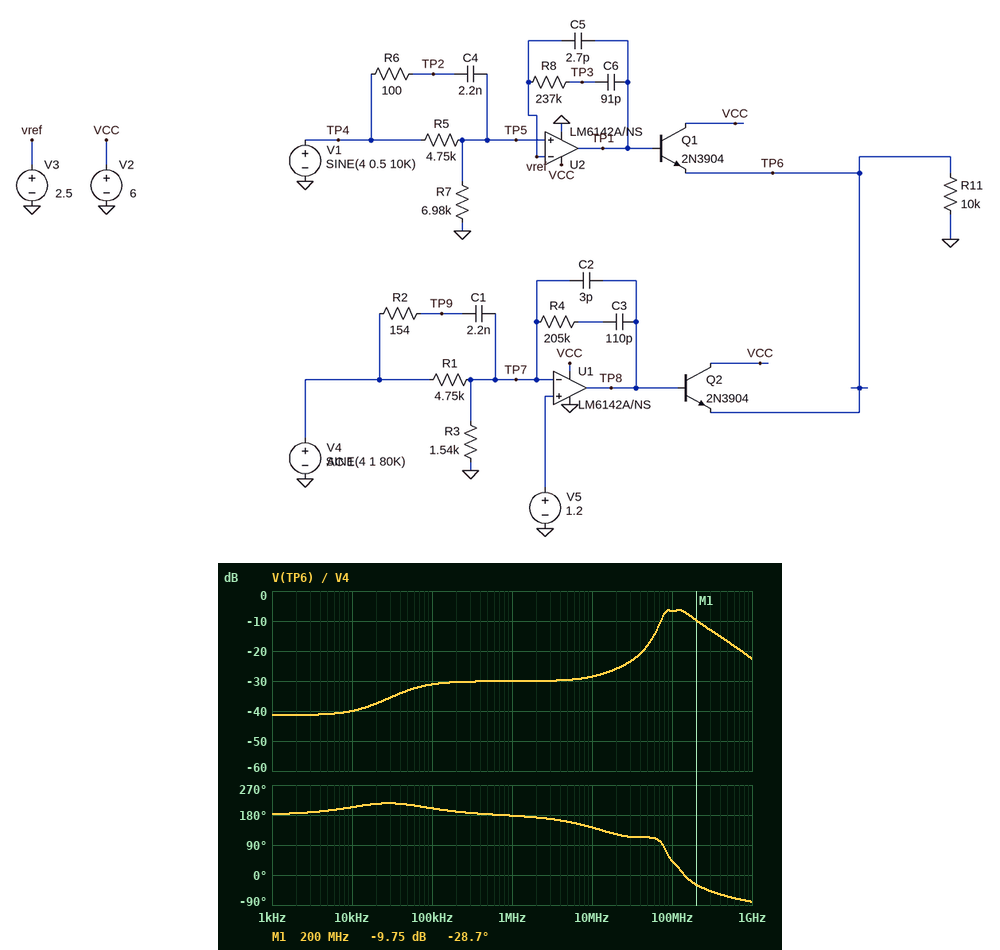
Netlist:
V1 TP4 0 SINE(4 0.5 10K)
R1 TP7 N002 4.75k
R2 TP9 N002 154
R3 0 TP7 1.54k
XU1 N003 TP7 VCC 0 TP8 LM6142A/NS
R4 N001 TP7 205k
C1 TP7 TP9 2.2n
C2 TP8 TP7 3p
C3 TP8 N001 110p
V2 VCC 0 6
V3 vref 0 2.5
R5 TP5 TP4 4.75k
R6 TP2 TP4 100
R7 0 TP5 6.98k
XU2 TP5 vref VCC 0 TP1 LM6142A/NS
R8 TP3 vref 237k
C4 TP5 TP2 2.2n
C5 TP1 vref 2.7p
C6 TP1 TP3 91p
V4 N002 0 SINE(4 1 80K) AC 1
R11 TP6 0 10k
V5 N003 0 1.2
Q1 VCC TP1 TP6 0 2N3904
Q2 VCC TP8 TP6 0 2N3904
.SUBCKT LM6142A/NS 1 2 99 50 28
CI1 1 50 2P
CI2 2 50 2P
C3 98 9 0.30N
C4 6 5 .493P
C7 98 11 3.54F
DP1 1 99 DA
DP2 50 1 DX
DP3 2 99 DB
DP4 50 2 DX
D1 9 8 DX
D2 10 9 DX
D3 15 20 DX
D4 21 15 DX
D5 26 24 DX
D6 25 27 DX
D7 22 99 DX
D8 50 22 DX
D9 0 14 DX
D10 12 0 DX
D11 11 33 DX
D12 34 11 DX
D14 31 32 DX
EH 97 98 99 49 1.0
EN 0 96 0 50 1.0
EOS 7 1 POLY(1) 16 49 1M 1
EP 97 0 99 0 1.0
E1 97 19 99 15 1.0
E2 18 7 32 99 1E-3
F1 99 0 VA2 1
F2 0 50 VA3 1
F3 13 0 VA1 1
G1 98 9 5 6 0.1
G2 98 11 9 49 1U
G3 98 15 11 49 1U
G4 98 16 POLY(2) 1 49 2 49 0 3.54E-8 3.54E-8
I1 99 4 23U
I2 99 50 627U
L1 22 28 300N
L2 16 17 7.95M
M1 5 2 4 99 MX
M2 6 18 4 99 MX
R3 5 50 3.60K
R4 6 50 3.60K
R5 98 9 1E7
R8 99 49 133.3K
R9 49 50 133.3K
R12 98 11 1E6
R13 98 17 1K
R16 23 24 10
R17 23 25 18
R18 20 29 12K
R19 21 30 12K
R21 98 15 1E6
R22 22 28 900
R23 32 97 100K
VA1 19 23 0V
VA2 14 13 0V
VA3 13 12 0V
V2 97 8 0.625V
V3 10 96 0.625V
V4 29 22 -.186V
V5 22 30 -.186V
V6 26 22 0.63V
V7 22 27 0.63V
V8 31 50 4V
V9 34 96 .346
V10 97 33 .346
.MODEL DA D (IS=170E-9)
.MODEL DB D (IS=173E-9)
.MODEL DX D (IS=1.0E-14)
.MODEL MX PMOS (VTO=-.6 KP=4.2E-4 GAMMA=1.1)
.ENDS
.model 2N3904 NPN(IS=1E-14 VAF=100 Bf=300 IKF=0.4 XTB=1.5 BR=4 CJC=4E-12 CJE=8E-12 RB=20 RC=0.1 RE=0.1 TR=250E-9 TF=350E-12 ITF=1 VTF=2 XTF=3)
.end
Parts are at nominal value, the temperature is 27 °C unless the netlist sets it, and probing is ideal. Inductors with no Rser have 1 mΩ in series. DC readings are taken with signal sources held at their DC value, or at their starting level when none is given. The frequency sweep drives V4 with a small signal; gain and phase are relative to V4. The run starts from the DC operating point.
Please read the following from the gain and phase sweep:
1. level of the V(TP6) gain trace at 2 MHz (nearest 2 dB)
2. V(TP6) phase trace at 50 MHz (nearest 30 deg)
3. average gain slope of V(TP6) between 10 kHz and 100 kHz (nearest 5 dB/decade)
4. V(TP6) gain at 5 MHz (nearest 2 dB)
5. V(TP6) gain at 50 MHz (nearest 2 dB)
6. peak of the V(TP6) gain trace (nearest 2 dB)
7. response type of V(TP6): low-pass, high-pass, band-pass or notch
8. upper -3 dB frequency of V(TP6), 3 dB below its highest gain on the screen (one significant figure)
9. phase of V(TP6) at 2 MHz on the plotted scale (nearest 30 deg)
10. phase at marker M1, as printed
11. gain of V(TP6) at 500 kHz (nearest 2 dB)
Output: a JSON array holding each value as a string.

["-30 dB", "120 deg", "10 dB/decade", "-30 dB", "-18 dB", "-6 dB", "band-pass", "200 MHz", "180 deg", "-28.7 deg", "-30 dB"]
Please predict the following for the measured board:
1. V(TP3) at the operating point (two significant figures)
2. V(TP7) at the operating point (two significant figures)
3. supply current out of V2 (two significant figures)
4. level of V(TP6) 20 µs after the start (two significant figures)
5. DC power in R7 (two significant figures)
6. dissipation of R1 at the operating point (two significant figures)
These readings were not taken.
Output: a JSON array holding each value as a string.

["2.5 V", "980 mV", "1.9 mA", "5.4 V", "810 µW", "1.9 mW"]
